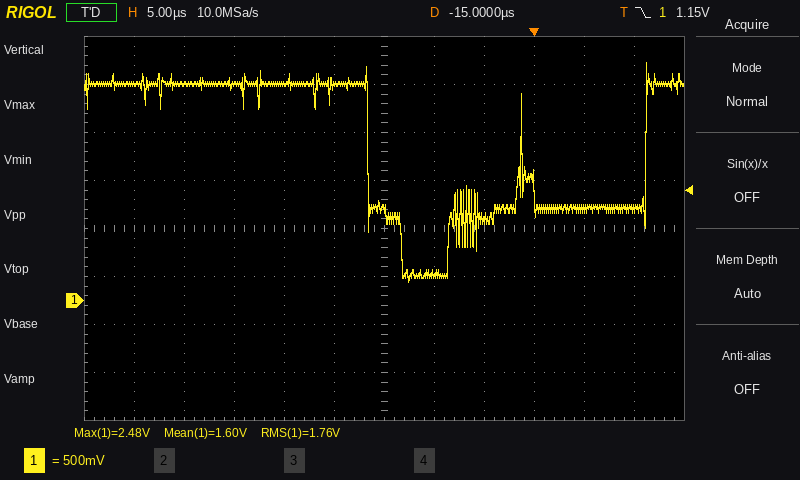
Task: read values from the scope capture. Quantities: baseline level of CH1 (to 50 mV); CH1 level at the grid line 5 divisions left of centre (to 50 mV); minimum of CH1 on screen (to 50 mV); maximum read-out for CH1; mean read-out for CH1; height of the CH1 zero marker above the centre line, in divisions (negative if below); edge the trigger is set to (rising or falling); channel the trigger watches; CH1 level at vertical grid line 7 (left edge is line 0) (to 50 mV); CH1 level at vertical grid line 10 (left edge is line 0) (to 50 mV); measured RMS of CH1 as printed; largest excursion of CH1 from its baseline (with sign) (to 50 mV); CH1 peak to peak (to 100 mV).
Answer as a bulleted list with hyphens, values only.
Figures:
- 2.25 V
- 2.25 V
- 200 mV
- 2.48 V
- 1.60 V
- -1.5 div
- falling
- CH1
- 300 mV
- 950 mV
- 1.76 V
- -2.05 V
- 2.30 V
